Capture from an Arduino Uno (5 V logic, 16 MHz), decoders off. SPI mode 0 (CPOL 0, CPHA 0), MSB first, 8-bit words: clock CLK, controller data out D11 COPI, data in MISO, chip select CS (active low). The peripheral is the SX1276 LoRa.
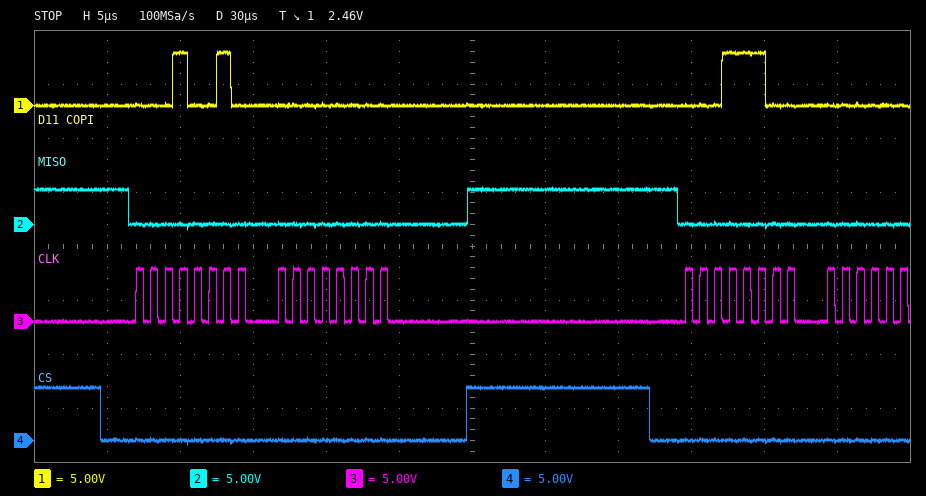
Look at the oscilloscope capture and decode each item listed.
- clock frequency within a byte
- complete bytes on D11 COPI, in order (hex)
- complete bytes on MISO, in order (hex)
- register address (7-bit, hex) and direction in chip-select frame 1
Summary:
1 MHz
12 00 1C
00 00 00
0x12 read
